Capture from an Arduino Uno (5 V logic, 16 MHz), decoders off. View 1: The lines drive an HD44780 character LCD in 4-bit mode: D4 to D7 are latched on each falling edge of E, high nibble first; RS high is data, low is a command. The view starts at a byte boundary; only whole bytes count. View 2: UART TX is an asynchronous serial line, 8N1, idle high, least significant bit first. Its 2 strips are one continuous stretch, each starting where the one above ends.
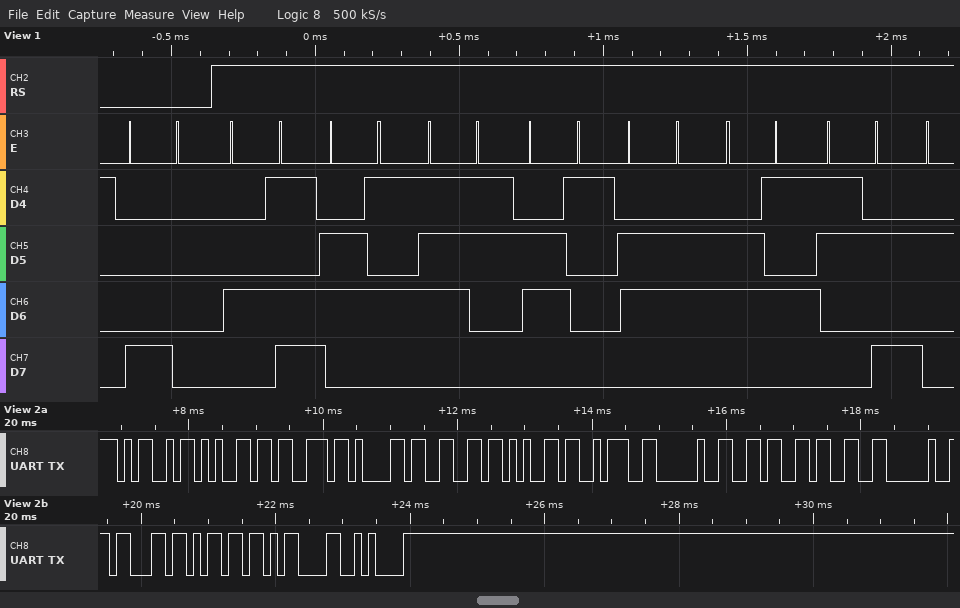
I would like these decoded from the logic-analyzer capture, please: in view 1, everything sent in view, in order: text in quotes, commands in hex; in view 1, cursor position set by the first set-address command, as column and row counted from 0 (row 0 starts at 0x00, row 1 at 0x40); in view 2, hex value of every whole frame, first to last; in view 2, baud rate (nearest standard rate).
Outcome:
0x80 "Mesafe:"
column 0, row 0
4D 65 73 61 66 65 3A 20 36 33 20 63 6D 0D 0A
9600 baud
